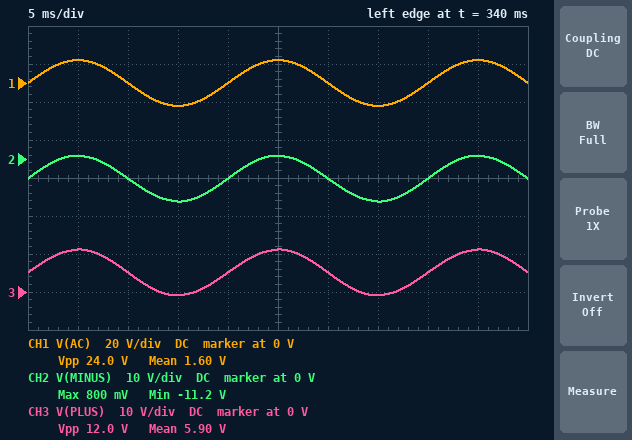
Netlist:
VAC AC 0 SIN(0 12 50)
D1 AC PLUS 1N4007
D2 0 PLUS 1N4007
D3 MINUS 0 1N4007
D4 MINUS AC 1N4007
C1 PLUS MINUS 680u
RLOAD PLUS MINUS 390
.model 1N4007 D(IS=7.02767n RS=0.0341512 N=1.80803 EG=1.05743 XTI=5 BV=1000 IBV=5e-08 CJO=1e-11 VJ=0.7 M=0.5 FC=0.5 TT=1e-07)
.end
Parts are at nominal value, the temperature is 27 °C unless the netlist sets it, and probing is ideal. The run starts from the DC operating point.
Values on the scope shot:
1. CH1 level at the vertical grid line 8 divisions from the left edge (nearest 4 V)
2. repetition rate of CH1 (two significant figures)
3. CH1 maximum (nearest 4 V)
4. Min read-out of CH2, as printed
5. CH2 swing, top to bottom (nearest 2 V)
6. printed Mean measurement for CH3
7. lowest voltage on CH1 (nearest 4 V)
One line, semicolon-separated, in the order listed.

0 V; 50 Hz; 12 V; -11.2 V; 12 V; 5.90 V; -12 V
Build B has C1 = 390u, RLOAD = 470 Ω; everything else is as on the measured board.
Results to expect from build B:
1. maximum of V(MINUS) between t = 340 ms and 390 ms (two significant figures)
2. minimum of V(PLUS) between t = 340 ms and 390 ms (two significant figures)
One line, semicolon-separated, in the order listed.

830 mV; -830 mV
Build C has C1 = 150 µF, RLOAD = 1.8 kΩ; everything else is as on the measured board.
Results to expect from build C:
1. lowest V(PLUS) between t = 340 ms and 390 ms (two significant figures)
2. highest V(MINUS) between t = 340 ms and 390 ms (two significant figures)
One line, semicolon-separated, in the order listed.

-760 mV; 760 mV
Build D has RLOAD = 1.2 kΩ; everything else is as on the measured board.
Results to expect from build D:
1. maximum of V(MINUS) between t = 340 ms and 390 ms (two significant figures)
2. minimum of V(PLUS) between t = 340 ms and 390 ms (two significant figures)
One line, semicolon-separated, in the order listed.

780 mV; -780 mV
